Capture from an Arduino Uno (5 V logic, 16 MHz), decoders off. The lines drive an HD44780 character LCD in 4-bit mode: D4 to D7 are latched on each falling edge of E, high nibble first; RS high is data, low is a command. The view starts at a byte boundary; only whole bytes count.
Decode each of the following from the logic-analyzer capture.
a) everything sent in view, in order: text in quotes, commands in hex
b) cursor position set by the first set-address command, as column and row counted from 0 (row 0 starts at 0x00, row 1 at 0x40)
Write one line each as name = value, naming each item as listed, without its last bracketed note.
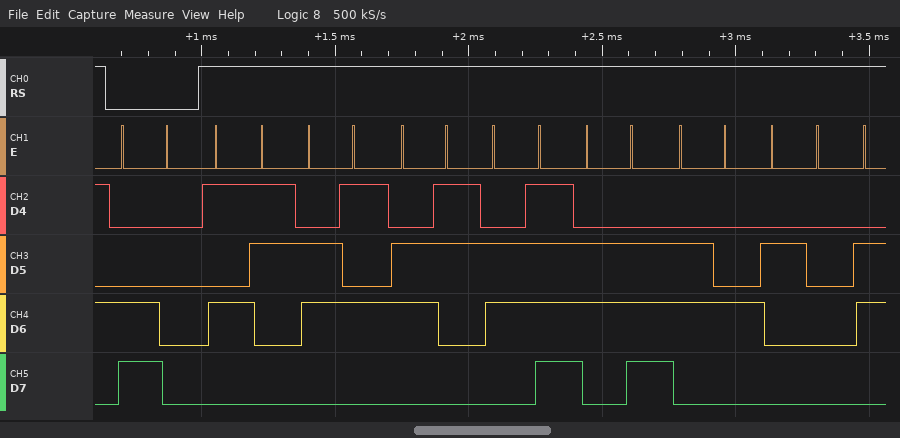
everything sent in view, in order: text in quotes, commands in hex = 0xC0 "Second "
cursor position set by the first set-address command, as column and row counted from 0 = column 0, row 1
